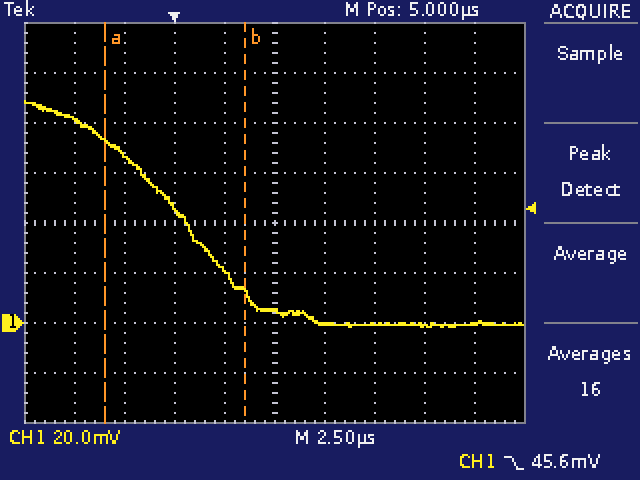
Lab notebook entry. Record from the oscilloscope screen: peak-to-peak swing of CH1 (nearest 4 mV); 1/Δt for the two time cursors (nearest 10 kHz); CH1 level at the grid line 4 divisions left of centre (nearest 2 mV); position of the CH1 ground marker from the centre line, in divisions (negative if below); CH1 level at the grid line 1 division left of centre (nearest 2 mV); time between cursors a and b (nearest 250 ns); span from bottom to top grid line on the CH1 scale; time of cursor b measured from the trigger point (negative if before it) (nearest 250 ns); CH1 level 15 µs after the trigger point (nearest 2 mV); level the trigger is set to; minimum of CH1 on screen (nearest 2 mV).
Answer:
92 mV
140 kHz
82 mV
-2.0 div
22 mV
7.00 µs
160 mV
+3.50 µs
0 mV
45.6 mV
-2 mV
